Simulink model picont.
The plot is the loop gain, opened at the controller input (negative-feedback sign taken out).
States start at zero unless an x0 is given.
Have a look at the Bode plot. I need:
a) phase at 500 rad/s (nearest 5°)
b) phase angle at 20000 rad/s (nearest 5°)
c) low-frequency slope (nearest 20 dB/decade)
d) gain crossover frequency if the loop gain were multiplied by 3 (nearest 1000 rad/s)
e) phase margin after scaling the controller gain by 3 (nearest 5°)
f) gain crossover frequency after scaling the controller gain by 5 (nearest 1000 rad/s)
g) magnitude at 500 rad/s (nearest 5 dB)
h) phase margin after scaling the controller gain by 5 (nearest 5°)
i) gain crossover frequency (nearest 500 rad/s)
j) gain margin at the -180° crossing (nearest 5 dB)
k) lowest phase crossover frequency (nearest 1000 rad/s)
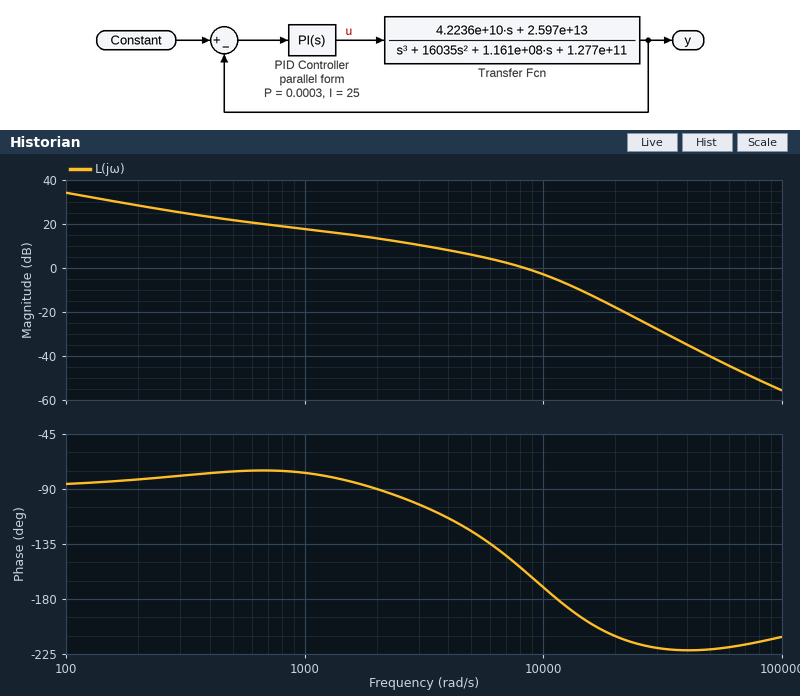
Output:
-75°
-210°
-20 dB/decade
14000 rad/s
-15°
17000 rad/s
20 dB
-25°
8500 rad/s
5 dB
11000 rad/s
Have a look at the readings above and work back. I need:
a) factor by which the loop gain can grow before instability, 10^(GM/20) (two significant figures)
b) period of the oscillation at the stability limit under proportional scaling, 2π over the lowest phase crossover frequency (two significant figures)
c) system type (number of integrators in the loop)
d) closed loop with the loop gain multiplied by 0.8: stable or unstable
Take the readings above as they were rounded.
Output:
1.8
0.00057 s
1
stable
